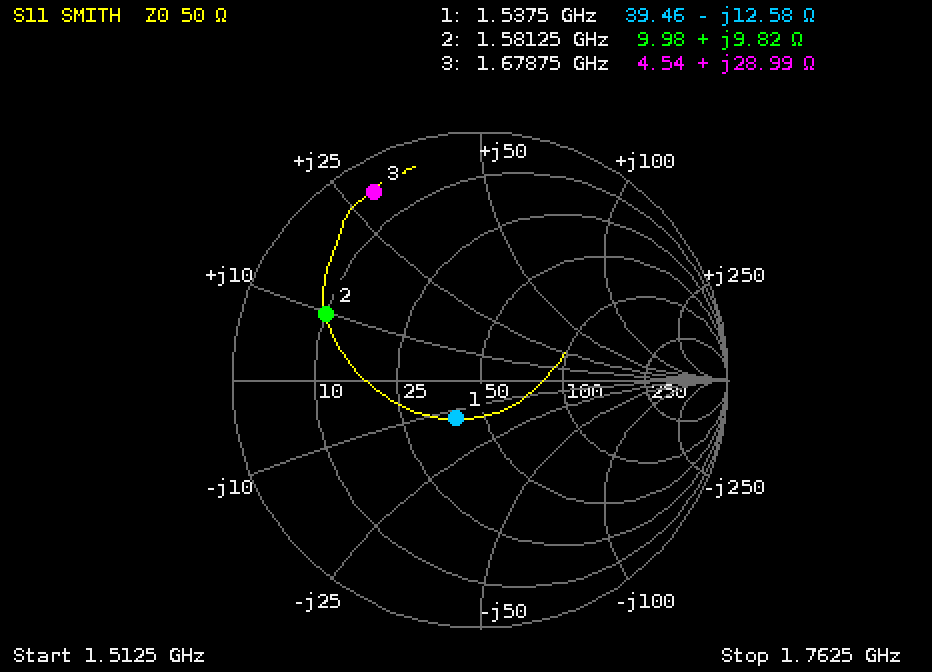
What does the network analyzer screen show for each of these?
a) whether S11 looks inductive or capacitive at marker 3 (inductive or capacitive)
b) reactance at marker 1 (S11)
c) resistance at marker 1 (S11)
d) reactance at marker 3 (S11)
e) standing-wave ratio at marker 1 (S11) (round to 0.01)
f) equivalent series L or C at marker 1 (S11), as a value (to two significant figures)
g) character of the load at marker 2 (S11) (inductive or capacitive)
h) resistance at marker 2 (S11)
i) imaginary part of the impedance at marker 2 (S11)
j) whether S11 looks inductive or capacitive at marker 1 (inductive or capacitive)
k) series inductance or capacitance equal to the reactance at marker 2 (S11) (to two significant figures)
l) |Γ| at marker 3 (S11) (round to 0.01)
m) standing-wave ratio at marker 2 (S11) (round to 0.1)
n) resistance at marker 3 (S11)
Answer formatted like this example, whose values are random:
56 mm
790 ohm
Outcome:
inductive
-12.58 Ω
39.46 Ω
+28.99 Ω
1.44
8.2 pF
inductive
9.98 Ω
+9.82 Ω
capacitive
990 pH
0.87
5.2
4.54 Ω
